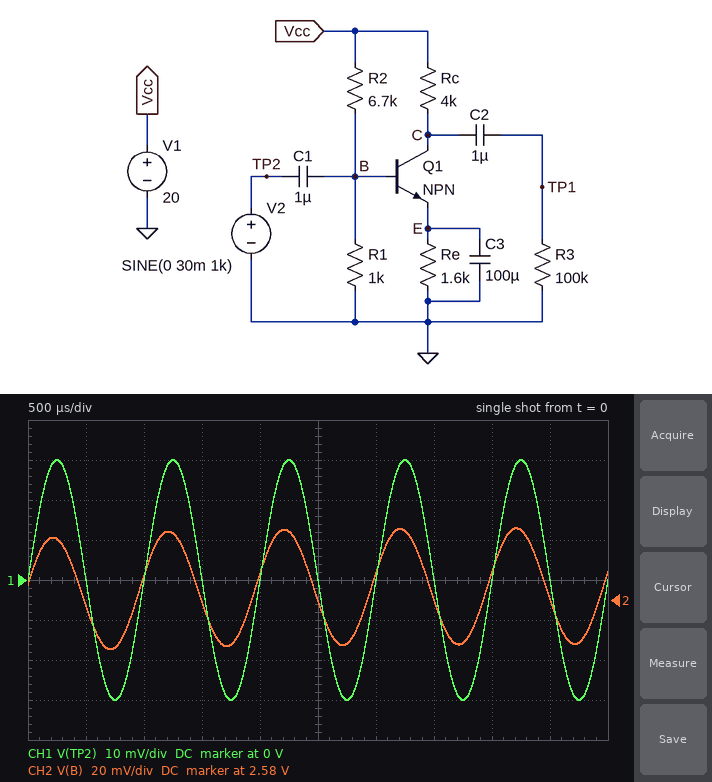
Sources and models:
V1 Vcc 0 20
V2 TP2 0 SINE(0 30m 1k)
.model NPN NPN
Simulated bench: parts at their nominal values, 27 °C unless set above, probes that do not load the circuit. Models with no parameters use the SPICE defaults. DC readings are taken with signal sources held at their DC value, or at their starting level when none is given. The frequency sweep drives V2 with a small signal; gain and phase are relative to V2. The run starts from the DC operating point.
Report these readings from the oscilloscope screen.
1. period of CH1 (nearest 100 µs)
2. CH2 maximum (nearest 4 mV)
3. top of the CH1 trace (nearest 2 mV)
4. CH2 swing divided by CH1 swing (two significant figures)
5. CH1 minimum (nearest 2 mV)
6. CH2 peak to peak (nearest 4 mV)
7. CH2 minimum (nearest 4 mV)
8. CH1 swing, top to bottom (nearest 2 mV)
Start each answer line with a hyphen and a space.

- 1.0 ms
- 2.616 V
- 30 mV
- 1.0
- -30 mV
- 60 mV
- 2.556 V
- 60 mV
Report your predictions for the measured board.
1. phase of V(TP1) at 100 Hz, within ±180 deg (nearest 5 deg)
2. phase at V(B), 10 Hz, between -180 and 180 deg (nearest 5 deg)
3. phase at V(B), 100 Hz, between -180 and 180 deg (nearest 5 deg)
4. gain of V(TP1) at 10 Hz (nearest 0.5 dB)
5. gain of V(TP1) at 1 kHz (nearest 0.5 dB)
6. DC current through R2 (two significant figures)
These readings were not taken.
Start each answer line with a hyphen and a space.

- -85 deg
- 85 deg
- 60 deg
- 2.0 dB
- 44.0 dB
- 2.6 mA
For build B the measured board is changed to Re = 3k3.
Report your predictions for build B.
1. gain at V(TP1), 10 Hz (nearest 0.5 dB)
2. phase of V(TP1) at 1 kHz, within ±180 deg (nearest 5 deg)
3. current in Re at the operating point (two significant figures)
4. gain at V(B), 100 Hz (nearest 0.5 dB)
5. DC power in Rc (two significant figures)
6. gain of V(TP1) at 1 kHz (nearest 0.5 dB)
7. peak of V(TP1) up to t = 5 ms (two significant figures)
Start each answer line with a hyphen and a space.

- 1.5 dB
- -165 deg
- 560 µA
- -7.5 dB
- 1.2 mW
- 38.0 dB
- 1.6 V
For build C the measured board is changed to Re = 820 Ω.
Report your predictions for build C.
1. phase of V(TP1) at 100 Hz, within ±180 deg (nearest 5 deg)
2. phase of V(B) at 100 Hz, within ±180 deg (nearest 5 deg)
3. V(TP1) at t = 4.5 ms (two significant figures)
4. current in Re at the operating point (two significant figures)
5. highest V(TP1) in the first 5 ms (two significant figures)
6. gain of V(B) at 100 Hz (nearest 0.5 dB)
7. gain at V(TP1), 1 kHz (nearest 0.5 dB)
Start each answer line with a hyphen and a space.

- -70 deg
- 55 deg
- 4.0 V
- 2.2 mA
- 6.1 V
- -9.0 dB
- 49.5 dB
